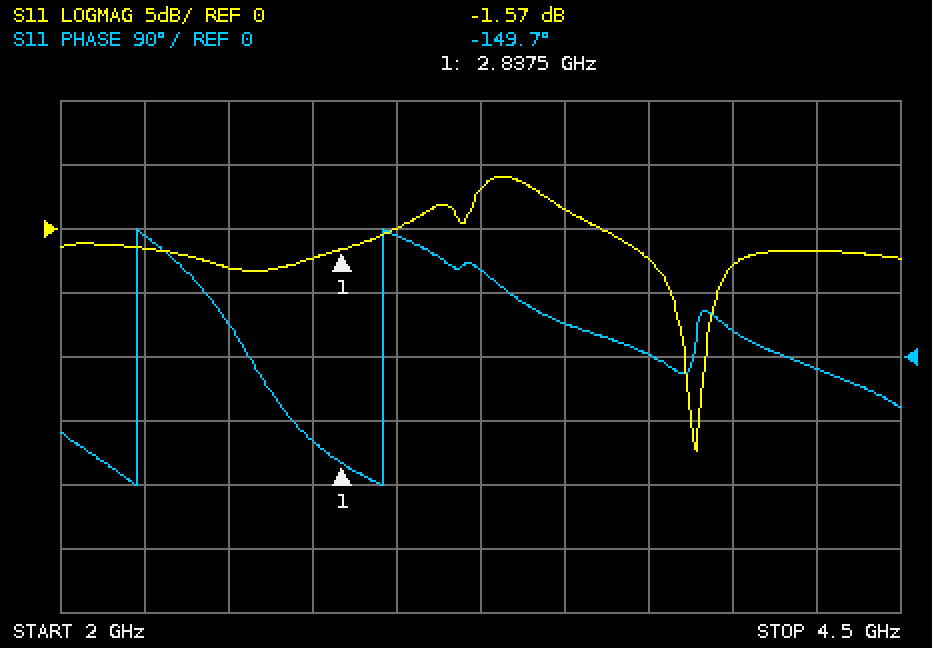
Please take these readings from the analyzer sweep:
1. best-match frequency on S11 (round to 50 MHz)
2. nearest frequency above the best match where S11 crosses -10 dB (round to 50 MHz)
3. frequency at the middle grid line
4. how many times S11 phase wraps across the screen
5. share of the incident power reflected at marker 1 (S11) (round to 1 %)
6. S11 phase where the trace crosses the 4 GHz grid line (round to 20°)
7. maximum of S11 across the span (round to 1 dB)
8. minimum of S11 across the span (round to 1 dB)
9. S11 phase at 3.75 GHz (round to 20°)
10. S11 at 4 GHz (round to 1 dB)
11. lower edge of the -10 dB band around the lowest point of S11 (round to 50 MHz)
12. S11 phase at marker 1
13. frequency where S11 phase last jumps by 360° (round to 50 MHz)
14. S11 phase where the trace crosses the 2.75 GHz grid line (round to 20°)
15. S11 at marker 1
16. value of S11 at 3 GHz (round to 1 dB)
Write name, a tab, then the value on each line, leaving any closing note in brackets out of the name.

best-match frequency on S11	3.90 GHz
nearest frequency above the best match where S11 crosses -10 dB	3.90 GHz
frequency at the middle grid line	3.25 GHz
how many times S11 phase wraps across the screen	2
share of the incident power reflected at marker 1 (S11)	70 %
S11 phase where the trace crosses the 4 GHz grid line	40°
maximum of S11 across the span	4 dB
minimum of S11 across the span	-17 dB
S11 phase at 3.75 GHz	0°
S11 at 4 GHz	-3 dB
lower edge of the -10 dB band around the lowest point of S11	3.85 GHz
S11 phase at marker 1	-149.7°
frequency where S11 phase last jumps by 360°	2.95 GHz
S11 phase where the trace crosses the 2.75 GHz grid line	-120°
S11 at marker 1	-1.57 dB
value of S11 at 3 GHz	0 dB
